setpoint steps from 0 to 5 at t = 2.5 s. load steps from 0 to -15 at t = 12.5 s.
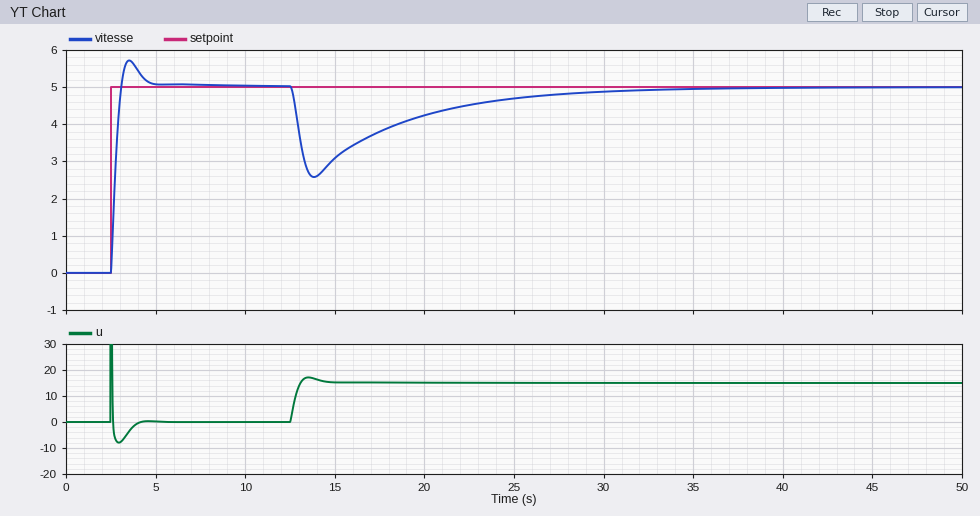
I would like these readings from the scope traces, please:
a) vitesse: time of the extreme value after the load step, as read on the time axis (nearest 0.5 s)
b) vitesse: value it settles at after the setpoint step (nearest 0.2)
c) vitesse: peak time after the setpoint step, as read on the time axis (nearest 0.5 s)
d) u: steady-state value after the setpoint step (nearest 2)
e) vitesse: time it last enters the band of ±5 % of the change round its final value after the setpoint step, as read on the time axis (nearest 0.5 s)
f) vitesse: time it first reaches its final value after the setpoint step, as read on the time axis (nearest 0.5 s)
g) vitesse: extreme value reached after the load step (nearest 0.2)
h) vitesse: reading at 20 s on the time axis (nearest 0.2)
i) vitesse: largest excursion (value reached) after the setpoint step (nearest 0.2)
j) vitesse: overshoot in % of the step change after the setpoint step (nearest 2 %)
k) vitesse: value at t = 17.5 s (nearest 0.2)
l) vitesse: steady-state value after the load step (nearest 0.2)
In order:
14.0 s
5.0
3.5 s
0
4.5 s
3.0 s
2.6
4.2
5.8
14 %
3.8
5.0
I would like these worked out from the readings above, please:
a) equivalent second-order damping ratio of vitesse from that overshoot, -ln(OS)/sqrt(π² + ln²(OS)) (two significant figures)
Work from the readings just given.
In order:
0.53
